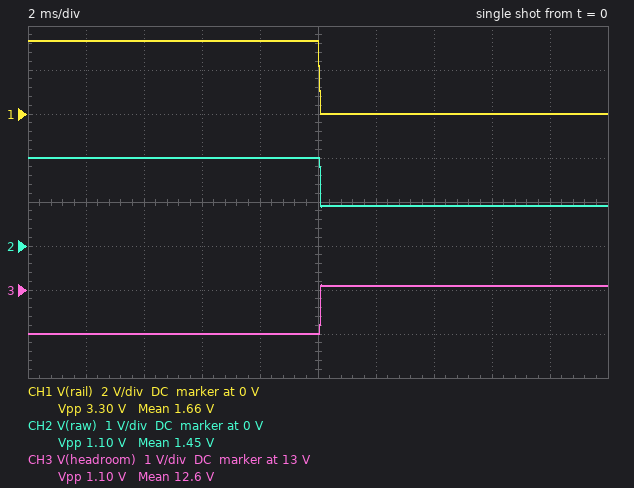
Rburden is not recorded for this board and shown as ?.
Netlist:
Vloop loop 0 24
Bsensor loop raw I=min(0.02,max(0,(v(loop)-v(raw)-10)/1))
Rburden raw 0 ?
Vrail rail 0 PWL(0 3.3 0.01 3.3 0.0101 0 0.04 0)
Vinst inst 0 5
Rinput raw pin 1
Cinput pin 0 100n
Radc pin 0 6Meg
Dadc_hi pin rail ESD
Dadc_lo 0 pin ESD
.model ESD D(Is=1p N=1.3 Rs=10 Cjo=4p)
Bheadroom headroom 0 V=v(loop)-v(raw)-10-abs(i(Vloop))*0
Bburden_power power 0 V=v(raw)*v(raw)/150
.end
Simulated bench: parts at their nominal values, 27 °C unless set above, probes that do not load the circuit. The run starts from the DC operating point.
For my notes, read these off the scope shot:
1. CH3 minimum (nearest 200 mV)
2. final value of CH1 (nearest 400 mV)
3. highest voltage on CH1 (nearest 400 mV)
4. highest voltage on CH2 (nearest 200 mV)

12.0 V
0 V
3.2 V
2.0 V
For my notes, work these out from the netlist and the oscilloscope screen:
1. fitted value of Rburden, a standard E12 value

100 Ω
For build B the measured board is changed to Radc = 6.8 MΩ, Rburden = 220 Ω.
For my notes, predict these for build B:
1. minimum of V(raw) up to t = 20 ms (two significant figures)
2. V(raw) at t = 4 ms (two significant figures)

960 mV
4.0 V
